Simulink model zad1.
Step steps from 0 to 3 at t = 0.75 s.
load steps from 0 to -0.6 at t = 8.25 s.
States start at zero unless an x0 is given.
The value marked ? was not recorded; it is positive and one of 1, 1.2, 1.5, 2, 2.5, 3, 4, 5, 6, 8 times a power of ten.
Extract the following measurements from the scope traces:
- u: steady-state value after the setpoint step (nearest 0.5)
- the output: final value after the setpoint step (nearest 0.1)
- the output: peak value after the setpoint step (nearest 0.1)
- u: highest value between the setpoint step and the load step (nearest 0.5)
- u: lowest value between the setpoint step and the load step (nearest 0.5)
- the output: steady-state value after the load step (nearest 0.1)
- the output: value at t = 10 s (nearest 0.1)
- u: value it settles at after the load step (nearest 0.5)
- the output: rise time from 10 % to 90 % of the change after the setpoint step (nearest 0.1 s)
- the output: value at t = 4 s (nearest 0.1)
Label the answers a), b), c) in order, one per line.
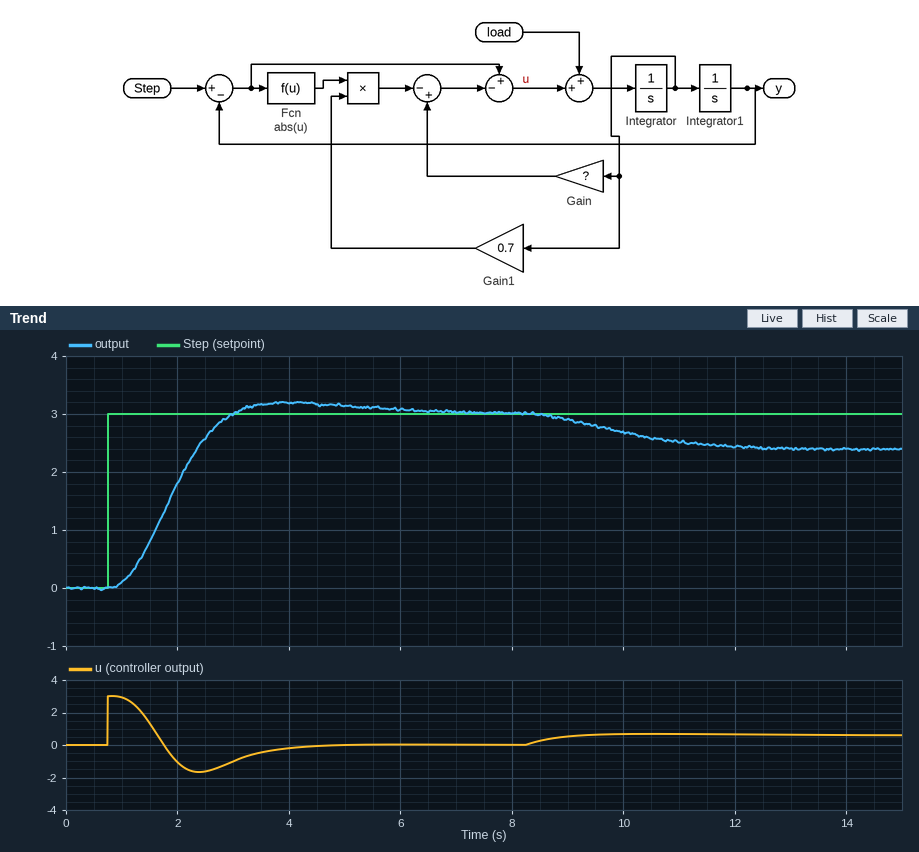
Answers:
a) 0.0
b) 3.0
c) 3.2
d) 3.0
e) -1.5
f) 2.4
g) 2.7
h) 0.5
i) 1.4 s
j) 3.2
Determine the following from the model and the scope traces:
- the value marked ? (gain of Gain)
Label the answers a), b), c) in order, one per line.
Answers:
a) 2
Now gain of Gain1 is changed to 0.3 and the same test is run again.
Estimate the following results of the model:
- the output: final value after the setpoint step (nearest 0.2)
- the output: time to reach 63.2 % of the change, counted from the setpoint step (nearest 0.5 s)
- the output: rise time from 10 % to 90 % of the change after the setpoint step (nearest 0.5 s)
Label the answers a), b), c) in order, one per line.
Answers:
a) 3.0
b) 1.5 s
c) 2.5 s
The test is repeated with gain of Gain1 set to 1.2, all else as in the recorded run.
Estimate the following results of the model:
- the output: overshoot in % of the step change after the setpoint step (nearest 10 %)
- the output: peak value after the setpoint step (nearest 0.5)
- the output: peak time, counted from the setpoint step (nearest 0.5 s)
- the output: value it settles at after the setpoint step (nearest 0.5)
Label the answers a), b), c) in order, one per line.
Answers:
a) 30 %
b) 4.0
c) 2.5 s
d) 3.0
